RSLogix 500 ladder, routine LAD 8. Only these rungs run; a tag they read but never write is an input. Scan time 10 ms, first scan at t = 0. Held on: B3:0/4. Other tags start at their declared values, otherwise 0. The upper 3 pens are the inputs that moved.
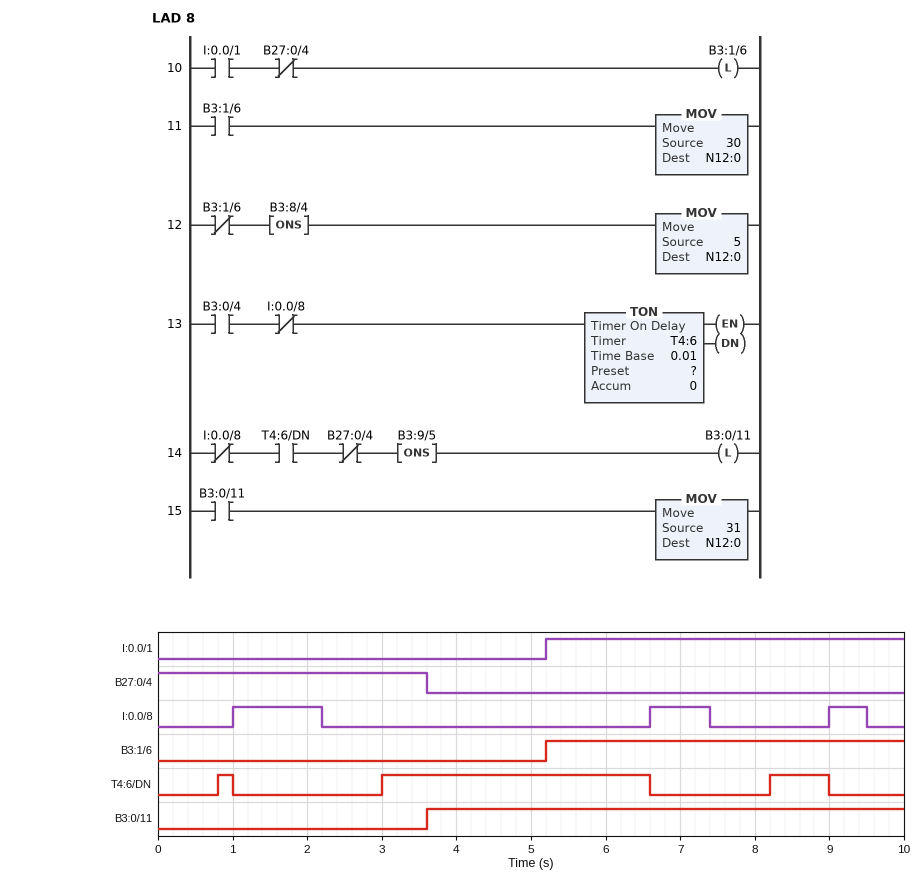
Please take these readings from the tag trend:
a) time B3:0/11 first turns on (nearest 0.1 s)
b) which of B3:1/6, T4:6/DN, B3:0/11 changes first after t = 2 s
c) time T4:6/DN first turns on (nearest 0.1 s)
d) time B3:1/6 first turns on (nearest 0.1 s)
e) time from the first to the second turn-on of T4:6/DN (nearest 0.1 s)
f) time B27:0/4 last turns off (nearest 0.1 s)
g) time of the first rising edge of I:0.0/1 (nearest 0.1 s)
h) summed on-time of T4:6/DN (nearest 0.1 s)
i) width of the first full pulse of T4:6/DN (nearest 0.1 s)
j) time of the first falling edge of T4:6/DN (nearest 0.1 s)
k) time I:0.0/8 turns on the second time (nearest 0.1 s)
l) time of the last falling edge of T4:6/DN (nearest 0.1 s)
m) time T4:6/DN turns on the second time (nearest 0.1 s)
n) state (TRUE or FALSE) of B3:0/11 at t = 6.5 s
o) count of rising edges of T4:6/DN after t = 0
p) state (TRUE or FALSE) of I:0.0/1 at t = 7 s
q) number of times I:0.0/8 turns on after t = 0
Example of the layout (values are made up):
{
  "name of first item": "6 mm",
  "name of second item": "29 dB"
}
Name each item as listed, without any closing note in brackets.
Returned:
{
  "time B3:0/11 first turns on": "3.6 s",
  "which of B3:1/6, T4:6/DN, B3:0/11 changes first after t = 2 s": "T4:6/DN",
  "time T4:6/DN first turns on": "0.8 s",
  "time B3:1/6 first turns on": "5.2 s",
  "time from the first to the second turn-on of T4:6/DN": "2.2 s",
  "time B27:0/4 last turns off": "3.6 s",
  "time of the first rising edge of I:0.0/1": "5.2 s",
  "summed on-time of T4:6/DN": "4.6 s",
  "width of the first full pulse of T4:6/DN": "0.2 s",
  "time of the first falling edge of T4:6/DN": "1.0 s",
  "time I:0.0/8 turns on the second time": "6.6 s",
  "time of the last falling edge of T4:6/DN": "9.0 s",
  "time T4:6/DN turns on the second time": "3.0 s",
  "state (TRUE or FALSE) of B3:0/11 at t = 6.5 s": "TRUE",
  "count of rising edges of T4:6/DN after t = 0": "3",
  "state (TRUE or FALSE) of I:0.0/1 at t = 7 s": "TRUE",
  "number of times I:0.0/8 turns on after t = 0": "3"
}
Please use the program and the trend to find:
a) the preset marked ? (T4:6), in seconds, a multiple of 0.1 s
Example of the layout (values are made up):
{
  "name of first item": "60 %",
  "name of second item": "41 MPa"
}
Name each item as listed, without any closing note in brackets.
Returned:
{
  "the preset marked ? (T4:6), in seconds, a multiple of 0.1 s": "0.8 s"
}
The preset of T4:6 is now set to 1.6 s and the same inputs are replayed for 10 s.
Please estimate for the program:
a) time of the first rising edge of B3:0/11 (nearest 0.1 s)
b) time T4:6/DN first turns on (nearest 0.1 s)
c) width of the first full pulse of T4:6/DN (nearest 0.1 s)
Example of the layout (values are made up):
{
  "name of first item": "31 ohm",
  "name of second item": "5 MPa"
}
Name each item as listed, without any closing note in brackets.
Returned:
{
  "time of the first rising edge of B3:0/11": "3.8 s",
  "time T4:6/DN first turns on": "3.8 s",
  "width of the first full pulse of T4:6/DN": "2.8 s"
}
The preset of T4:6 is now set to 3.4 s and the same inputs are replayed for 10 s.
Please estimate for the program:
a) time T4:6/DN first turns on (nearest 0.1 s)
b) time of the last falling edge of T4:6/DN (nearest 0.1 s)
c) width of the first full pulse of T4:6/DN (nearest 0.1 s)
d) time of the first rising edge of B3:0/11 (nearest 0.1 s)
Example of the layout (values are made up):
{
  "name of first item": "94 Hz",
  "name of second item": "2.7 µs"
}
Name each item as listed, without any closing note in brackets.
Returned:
{
  "time T4:6/DN first turns on": "5.6 s",
  "time of the last falling edge of T4:6/DN": "6.6 s",
  "width of the first full pulse of T4:6/DN": "1.0 s",
  "time of the first rising edge of B3:0/11": "5.6 s"
}
